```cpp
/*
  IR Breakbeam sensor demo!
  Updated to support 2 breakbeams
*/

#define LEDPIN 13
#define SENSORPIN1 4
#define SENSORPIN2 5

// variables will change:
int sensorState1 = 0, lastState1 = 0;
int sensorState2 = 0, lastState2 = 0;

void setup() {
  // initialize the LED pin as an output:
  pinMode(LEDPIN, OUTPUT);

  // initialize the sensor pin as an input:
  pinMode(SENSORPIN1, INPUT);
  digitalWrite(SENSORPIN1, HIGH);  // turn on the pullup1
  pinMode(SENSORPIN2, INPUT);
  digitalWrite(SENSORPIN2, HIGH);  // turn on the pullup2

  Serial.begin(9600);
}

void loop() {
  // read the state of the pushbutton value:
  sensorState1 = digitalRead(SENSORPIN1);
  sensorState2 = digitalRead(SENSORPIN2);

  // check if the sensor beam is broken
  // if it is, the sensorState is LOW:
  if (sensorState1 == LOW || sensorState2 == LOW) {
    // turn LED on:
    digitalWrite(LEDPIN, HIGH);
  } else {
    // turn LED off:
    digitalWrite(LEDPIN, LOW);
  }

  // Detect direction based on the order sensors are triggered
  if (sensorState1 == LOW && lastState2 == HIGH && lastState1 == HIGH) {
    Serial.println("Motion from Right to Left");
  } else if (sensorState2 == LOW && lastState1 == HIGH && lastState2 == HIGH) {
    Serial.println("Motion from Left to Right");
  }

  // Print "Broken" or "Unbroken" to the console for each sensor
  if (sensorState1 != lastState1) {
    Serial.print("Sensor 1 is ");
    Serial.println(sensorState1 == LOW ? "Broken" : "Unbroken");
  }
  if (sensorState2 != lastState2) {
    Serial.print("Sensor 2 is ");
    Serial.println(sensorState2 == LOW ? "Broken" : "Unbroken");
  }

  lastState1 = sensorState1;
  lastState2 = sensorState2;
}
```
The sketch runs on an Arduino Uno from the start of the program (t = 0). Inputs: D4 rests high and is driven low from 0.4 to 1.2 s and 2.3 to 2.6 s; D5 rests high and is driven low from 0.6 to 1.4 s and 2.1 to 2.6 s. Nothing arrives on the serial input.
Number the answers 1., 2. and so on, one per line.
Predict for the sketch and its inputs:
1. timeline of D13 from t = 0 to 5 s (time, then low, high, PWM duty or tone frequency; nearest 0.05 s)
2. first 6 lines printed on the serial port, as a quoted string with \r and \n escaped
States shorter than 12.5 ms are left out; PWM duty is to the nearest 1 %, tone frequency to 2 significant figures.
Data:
1. 0 s low; 0.4 s high; 1.4 s low; 2.1 s high; 2.6 s low
2. "Sensor 1 is Unbroken\r\nSensor 2 is Unbroken\r\nMotion from Right to Left\r\nSensor 1 is Broken\r\nSensor 2 is Broken\r\nSensor 1 is Unbroken\r\n"
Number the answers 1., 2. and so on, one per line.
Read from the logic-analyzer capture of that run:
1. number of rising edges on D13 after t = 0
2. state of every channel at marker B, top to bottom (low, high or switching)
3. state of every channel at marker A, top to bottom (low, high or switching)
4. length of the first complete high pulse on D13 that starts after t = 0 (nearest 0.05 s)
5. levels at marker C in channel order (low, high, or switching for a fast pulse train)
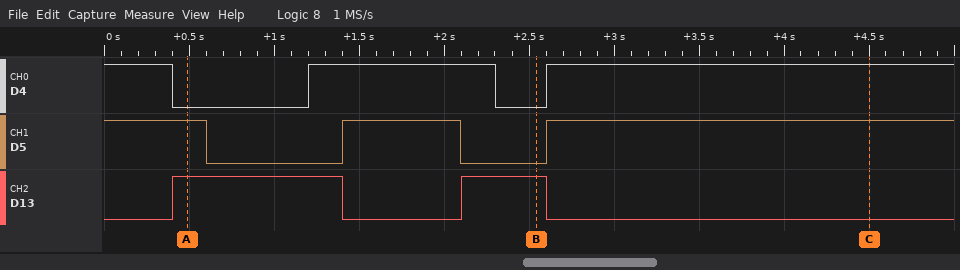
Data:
1. 2
2. D4 low, D5 low, D13 high
3. D4 low, D5 high, D13 high
4. 1.00 s
5. D4 high, D5 high, D13 low
